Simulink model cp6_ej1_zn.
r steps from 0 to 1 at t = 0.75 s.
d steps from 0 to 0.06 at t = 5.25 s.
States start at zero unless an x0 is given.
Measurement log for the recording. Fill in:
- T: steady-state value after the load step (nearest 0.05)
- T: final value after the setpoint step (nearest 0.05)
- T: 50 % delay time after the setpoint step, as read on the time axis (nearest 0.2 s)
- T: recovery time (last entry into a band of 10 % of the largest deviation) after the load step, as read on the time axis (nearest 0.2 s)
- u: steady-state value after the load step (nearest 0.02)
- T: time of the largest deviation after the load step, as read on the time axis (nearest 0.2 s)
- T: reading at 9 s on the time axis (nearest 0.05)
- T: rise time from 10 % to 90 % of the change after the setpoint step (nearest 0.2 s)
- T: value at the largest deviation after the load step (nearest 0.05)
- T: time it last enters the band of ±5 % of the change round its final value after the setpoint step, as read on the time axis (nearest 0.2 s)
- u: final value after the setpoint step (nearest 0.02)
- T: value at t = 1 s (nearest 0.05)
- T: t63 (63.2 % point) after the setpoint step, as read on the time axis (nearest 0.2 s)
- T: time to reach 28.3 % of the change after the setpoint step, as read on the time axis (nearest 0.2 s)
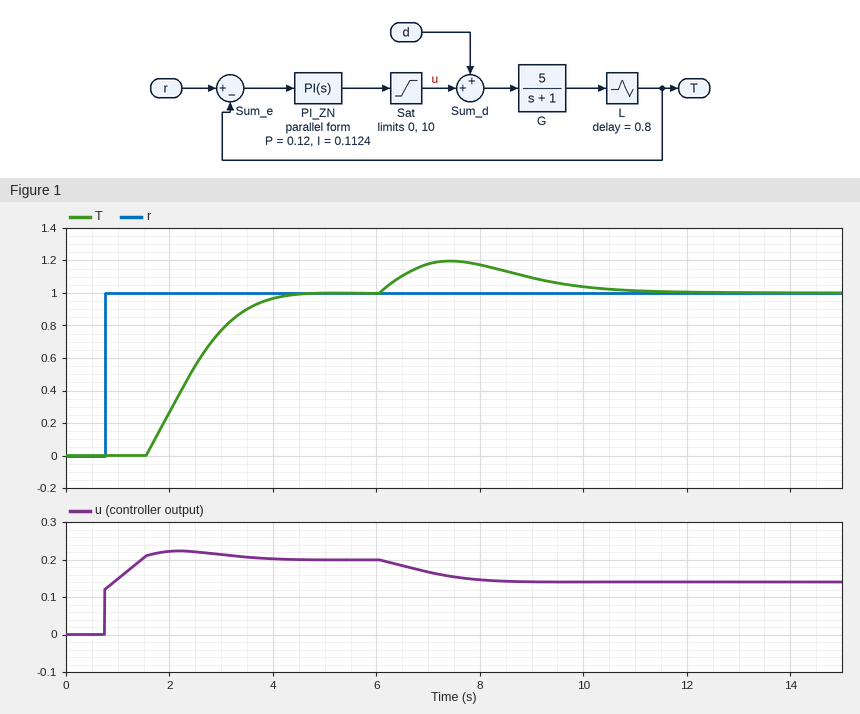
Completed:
1.00
1.00
2.4 s
10.6 s
0.14
7.4 s
1.10
1.8 s
1.20
3.8 s
0.20
0.00
2.6 s
2.0 s
